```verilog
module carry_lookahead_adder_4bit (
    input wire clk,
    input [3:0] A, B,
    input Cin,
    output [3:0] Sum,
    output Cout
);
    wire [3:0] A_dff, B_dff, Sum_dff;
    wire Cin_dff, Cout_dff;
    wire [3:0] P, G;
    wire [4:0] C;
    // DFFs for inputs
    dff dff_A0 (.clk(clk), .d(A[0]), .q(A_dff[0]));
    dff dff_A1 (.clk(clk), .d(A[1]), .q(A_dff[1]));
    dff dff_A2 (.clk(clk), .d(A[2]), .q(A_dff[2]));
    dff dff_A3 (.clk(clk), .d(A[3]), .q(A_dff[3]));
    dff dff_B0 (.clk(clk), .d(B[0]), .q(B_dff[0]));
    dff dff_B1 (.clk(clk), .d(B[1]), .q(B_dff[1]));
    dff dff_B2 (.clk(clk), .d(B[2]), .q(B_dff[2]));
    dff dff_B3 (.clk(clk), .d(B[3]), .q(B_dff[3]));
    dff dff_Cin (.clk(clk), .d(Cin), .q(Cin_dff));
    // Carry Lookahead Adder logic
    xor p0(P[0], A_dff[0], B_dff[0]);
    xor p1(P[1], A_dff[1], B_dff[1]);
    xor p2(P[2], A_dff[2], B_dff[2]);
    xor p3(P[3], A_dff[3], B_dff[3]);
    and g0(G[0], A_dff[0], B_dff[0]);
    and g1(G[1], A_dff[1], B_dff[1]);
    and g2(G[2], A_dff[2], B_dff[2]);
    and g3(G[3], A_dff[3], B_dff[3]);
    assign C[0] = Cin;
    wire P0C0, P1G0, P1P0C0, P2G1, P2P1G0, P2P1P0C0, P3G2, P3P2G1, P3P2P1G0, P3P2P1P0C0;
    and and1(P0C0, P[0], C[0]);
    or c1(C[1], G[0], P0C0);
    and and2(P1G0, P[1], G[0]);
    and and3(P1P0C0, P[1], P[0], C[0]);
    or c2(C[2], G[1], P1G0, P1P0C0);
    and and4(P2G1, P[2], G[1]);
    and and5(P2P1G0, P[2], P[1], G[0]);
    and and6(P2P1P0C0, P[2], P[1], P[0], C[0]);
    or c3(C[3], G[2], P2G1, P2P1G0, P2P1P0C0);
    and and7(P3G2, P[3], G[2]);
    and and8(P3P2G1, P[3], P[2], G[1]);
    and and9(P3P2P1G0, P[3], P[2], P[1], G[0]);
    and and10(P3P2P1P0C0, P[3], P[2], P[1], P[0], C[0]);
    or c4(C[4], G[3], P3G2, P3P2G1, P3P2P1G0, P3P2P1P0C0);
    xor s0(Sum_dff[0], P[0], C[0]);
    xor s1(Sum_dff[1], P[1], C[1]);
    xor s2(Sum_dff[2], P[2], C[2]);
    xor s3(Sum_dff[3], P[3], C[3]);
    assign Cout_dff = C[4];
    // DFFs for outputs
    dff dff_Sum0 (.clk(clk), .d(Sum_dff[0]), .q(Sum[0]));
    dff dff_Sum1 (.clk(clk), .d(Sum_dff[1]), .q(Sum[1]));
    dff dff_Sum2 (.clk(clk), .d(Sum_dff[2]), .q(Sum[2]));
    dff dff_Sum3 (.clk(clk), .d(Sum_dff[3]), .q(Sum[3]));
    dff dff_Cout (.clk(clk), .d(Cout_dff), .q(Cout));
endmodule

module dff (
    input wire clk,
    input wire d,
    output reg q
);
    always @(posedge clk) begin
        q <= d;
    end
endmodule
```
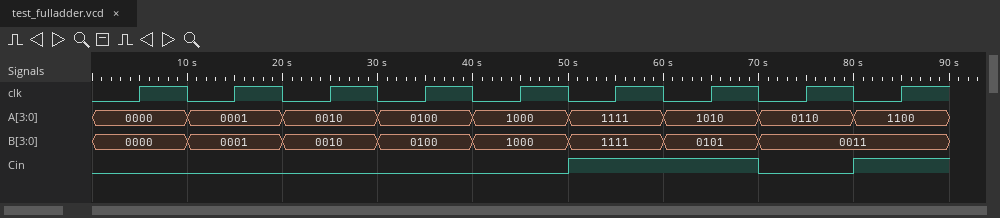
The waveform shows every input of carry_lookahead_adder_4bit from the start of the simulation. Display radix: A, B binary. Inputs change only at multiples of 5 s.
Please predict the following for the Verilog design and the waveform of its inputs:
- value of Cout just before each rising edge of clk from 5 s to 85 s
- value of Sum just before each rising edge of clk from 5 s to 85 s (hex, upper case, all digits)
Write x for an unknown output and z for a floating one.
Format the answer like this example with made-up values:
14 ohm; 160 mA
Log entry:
x x 0 0 0 0 1 1 0; x, x, 0, 2, 4, 8, 1, F, F
